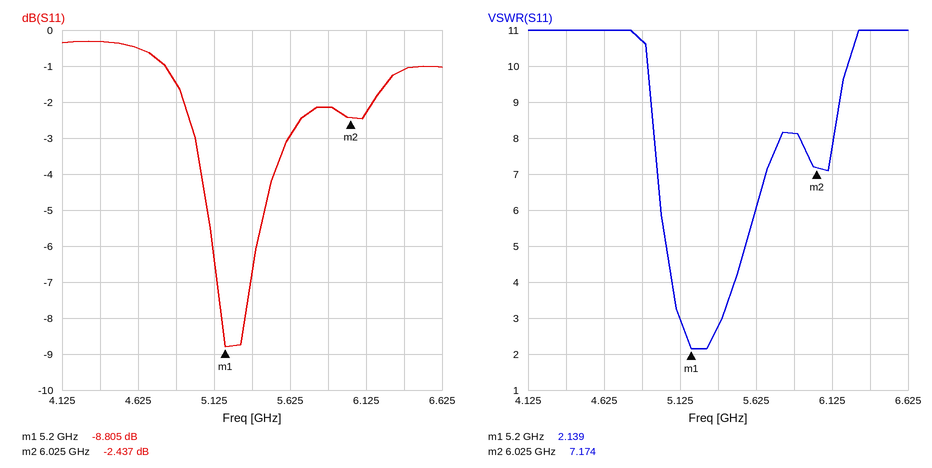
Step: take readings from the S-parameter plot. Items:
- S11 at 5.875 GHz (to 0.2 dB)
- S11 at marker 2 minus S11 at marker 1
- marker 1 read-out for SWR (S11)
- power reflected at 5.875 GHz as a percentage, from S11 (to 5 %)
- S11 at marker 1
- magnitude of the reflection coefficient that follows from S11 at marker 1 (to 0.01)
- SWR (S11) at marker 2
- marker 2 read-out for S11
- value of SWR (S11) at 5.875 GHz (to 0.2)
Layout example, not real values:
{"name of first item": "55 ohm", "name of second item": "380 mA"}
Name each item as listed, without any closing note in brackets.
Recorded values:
{"S11 at 5.875 GHz": "-2.2 dB", "S11 at marker 2 minus S11 at marker 1": "6.368 dB", "marker 1 read-out for SWR": "2.139", "power reflected at 5.875 GHz as a percentage, from S11": "60 %", "S11 at marker 1": "-8.805 dB", "magnitude of the reflection coefficient that follows from S11 at marker 1": "0.36", "SWR (S11) at marker 2": "7.174", "marker 2 read-out for S11": "-2.437 dB", "value of SWR (S11) at 5.875 GHz": "8.2"}
